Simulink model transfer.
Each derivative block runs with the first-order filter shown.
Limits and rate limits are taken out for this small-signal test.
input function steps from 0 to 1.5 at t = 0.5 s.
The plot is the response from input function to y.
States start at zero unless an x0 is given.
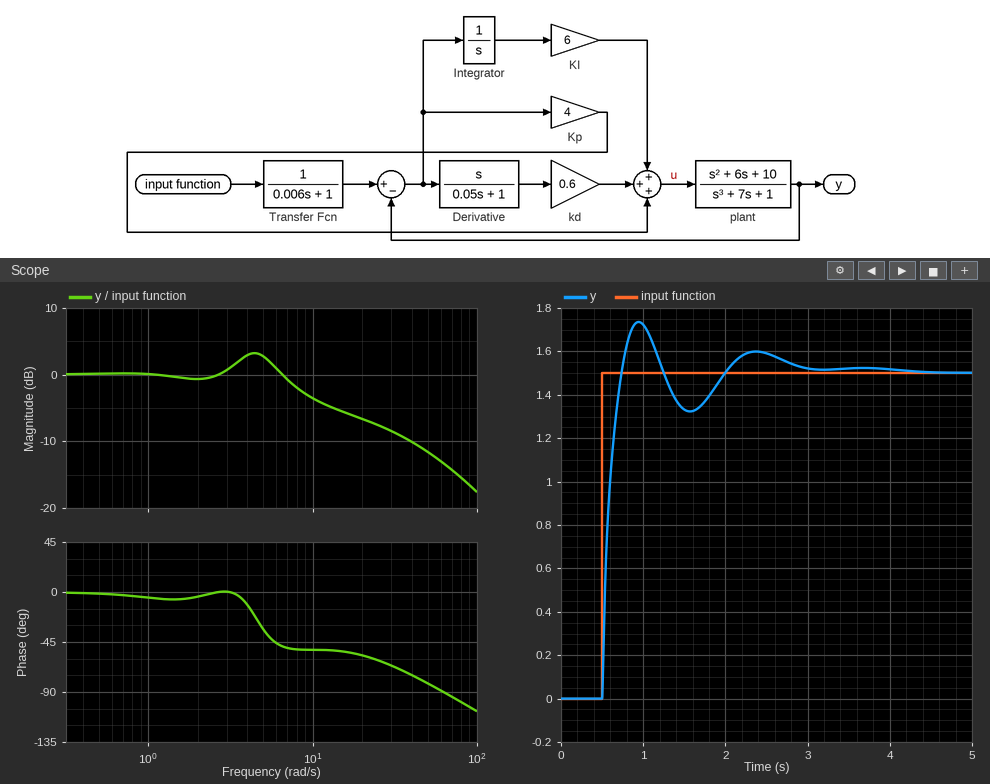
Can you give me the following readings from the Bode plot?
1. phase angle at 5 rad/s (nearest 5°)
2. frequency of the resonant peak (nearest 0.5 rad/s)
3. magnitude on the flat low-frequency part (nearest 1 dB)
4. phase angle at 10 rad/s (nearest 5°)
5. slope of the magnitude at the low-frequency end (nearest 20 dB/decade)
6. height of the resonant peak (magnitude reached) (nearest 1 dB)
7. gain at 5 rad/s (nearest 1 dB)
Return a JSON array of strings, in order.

["-35°", "4.5 rad/s", "0 dB", "-50°", "0 dB/decade", "3 dB", "3 dB"]
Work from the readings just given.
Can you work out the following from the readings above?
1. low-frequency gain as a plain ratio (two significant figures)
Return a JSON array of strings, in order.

["1.0"]
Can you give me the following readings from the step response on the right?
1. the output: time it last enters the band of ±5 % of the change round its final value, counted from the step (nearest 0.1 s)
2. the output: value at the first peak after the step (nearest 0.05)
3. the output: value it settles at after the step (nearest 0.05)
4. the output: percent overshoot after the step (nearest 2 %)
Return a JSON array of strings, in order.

["2.1 s", "1.75", "1.50", "16 %"]
